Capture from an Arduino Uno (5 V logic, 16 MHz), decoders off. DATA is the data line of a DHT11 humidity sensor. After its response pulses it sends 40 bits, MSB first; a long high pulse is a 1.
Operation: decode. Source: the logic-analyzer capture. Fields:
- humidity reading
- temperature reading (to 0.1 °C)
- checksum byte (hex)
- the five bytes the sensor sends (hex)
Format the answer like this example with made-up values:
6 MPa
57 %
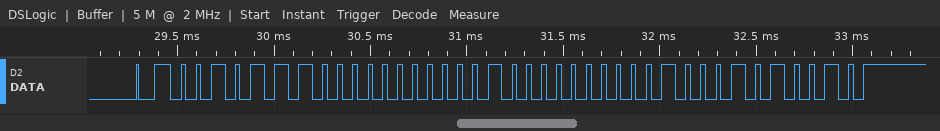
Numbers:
46 %
32.4 °C
0x52
2E 00 20 04 52
